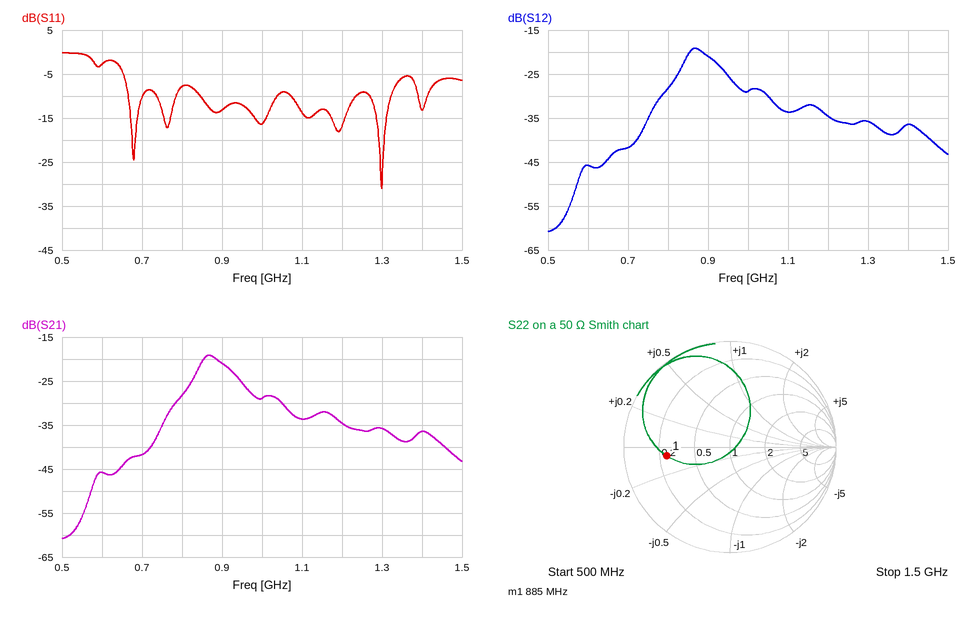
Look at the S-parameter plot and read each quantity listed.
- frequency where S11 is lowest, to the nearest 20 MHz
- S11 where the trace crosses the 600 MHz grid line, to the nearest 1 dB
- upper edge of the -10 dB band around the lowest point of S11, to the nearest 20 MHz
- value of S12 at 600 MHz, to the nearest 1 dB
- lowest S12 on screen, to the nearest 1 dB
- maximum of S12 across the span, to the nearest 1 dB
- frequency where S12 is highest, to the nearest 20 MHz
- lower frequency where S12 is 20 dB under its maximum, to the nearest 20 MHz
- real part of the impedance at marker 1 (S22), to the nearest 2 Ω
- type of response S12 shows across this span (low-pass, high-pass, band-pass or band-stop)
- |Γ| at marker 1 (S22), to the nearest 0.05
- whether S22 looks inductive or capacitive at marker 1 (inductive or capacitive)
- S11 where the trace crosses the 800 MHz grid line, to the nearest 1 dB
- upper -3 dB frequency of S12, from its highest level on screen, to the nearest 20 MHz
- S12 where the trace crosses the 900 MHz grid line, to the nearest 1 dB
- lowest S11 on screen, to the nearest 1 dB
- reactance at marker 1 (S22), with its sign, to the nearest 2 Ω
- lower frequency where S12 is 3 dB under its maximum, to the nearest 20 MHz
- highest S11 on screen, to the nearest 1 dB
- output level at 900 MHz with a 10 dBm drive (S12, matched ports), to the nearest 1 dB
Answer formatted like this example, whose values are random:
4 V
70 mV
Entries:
1.30 GHz
-3 dB
1.32 GHz
-46 dB
-61 dB
-19 dB
860 MHz
720 MHz
12 Ω
band-pass
0.60
capacitive
-8 dB
920 MHz
-21 dB
-31 dB
-4 Ω
840 MHz
0 dB
-11 dBm
